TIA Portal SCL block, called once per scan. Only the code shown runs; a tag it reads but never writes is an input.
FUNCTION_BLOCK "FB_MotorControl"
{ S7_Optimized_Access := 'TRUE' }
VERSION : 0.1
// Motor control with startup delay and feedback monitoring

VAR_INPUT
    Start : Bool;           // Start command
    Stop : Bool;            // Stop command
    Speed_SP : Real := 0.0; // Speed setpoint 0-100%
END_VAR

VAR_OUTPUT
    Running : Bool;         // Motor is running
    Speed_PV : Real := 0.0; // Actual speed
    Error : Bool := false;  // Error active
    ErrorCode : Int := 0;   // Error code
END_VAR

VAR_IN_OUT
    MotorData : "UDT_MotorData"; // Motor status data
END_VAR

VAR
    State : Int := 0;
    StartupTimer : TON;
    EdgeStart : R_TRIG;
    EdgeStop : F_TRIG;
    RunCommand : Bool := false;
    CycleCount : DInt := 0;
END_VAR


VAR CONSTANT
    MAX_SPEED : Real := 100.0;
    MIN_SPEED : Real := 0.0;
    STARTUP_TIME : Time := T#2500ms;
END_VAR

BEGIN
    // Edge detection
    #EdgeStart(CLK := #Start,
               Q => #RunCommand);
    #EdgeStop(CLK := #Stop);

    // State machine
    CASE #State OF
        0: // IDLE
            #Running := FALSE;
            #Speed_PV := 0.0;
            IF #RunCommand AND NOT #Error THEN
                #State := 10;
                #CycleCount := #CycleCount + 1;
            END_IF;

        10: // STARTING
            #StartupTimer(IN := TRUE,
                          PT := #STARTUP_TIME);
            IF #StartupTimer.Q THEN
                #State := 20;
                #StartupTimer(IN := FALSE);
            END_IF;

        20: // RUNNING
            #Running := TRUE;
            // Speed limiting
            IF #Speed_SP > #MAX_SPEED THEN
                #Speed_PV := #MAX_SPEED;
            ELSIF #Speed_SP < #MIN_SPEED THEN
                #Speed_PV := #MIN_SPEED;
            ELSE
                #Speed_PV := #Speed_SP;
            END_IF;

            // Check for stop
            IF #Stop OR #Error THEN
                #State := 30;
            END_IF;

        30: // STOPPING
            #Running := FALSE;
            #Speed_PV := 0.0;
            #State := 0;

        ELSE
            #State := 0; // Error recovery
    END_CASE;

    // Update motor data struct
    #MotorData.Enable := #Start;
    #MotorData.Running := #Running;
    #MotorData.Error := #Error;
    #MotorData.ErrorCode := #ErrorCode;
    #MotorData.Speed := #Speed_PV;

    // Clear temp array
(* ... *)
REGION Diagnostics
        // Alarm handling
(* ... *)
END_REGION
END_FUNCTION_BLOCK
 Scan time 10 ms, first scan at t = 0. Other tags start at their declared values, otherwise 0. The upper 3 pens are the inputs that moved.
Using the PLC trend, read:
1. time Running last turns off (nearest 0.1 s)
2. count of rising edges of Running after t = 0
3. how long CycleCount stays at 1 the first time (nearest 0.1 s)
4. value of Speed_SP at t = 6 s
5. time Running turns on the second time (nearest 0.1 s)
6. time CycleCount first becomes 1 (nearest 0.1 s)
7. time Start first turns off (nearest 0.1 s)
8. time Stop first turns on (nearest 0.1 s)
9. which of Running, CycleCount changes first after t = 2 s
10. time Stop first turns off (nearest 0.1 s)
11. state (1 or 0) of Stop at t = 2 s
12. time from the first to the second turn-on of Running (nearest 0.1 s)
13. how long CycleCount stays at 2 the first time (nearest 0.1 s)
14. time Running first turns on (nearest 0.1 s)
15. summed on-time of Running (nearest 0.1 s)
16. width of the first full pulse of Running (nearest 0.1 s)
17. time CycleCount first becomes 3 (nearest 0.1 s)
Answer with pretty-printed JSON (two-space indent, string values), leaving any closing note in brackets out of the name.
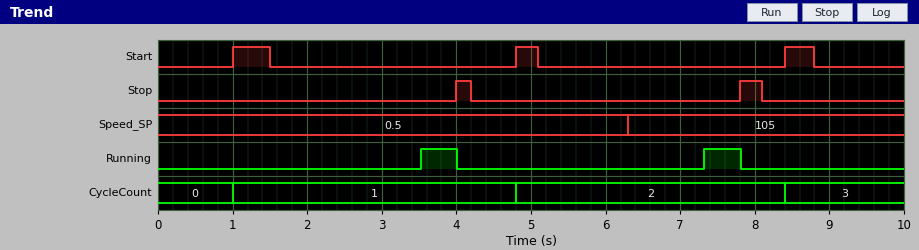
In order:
{
  "time Running last turns off": "7.8 s",
  "count of rising edges of Running after t = 0": "2",
  "how long CycleCount stays at 1 the first time": "3.8 s",
  "value of Speed_SP at t = 6 s": "0.5",
  "time Running turns on the second time": "7.3 s",
  "time CycleCount first becomes 1": "1.0 s",
  "time Start first turns off": "1.5 s",
  "time Stop first turns on": "4.0 s",
  "which of Running, CycleCount changes first after t = 2 s": "Running",
  "time Stop first turns off": "4.2 s",
  "state (1 or 0) of Stop at t = 2 s": "0",
  "time from the first to the second turn-on of Running": "3.8 s",
  "how long CycleCount stays at 2 the first time": "3.6 s",
  "time Running first turns on": "3.5 s",
  "summed on-time of Running": "1.0 s",
  "width of the first full pulse of Running": "0.5 s",
  "time CycleCount first becomes 3": "8.4 s"
}
